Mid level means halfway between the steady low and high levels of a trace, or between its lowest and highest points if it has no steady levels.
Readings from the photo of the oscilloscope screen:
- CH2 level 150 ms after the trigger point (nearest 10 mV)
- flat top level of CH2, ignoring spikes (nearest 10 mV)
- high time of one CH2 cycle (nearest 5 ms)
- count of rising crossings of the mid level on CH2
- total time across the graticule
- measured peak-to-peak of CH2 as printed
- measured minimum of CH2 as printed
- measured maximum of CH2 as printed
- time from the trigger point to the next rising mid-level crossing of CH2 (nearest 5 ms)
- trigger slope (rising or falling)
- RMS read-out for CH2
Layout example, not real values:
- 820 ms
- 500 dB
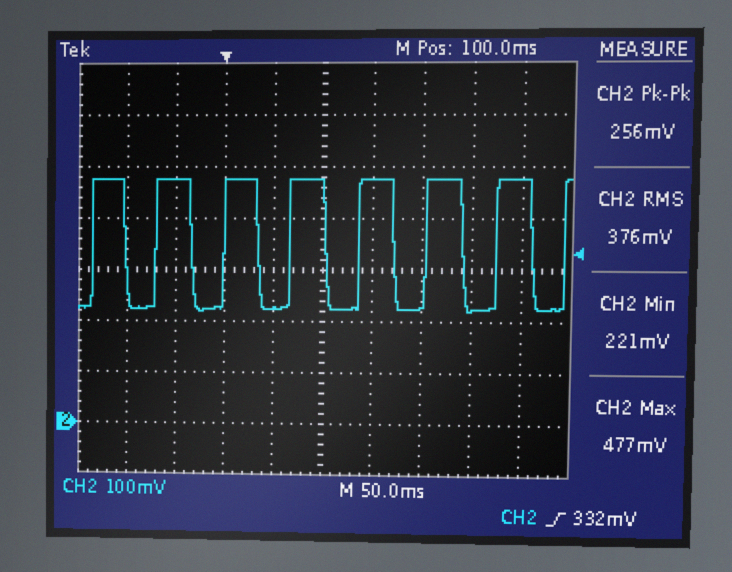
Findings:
- 480 mV
- 480 mV
- 35 ms
- 8
- 500 ms
- 256 mV
- 221 mV
- 477 mV
- 65 ms
- rising
- 376 mV
